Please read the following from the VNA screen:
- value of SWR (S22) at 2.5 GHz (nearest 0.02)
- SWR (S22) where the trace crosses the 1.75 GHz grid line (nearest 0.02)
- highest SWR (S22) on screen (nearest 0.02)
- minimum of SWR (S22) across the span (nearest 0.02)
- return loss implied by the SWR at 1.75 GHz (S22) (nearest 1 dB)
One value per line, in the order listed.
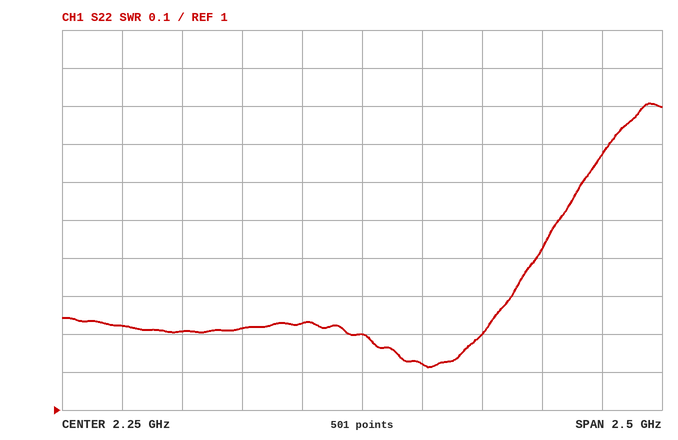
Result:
1.12
1.22
1.80
1.12
20 dB
